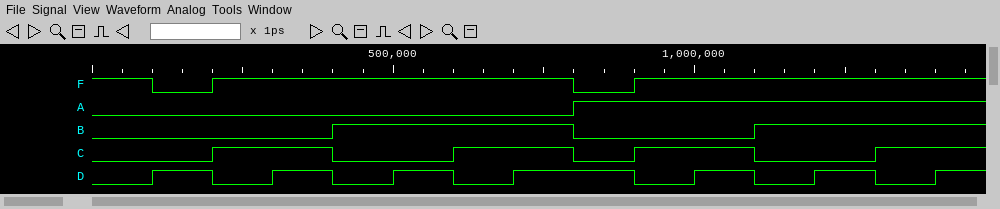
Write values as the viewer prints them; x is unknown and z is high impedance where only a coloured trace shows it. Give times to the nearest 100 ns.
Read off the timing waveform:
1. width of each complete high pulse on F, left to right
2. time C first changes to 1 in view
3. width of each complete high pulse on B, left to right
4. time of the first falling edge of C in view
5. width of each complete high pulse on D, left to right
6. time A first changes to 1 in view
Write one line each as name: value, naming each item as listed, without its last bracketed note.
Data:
width of each complete high pulse on F, left to right: 600 ns
time C first changes to 1 in view: 200 ns
width of each complete high pulse on B, left to right: 400 ns
time of the first falling edge of C in view: 400 ns
width of each complete high pulse on D, left to right: 100 ns, 100 ns, 100 ns, 200 ns, 100 ns, 100 ns
time A first changes to 1 in view: 800 ns
